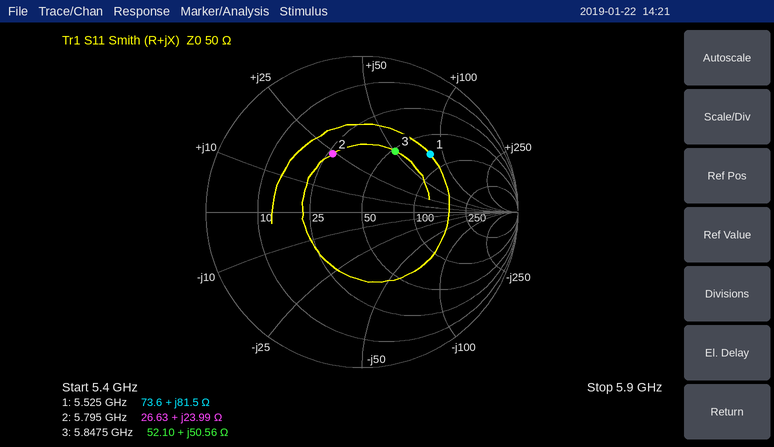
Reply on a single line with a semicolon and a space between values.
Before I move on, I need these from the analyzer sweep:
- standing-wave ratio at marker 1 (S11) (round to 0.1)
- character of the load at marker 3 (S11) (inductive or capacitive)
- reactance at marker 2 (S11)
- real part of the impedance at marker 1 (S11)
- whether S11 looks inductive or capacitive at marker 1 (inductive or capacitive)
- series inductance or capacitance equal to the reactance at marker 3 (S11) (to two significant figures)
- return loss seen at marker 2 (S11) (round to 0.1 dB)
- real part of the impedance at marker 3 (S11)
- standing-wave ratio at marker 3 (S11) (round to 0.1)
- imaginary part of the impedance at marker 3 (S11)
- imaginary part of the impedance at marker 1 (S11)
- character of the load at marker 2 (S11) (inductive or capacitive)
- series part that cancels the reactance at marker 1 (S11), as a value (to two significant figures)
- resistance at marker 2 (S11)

3.7; inductive; +23.99 Ω; 73.6 Ω; inductive; 1.4 nH; 7.6 dB; 52.10 Ω; 2.6; +50.56 Ω; +81.5 Ω; inductive; 350 fF; 26.63 Ω
